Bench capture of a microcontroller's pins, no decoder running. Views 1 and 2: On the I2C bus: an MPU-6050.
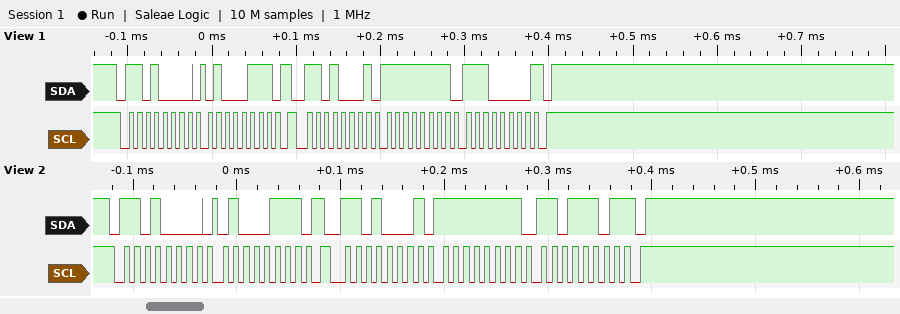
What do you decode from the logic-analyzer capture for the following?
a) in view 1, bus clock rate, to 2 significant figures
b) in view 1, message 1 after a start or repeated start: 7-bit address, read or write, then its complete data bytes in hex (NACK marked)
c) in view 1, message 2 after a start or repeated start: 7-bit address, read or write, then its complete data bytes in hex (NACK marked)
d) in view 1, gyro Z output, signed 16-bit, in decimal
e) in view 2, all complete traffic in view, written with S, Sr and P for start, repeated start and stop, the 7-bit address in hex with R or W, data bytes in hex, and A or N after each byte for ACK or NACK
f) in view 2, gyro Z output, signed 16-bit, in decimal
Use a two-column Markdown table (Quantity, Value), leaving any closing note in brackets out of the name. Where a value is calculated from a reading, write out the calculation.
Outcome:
| Quantity | Value |
|---|---|
| in view 1, bus clock rate, to 2 significant figures | 100 kHz |
| in view 1, message 1 after a start or repeated start: 7-bit address, read or write, then its complete data bytes in hex | 0x68 write: 47 |
| in view 1, message 2 after a start or repeated start: 7-bit address, read or write, then its complete data bytes in hex | 0x68 read: FF E0 NACK |
| in view 1, gyro Z output, signed 16-bit, in decimal | 0xFFE0 = -32 |
| in view 2, all complete traffic in view, written with S, Sr and P for start, repeated start and stop, the 7-bit address in hex with R or W, data bytes in hex, and A or N after each byte for ACK or NACK | S 68W A 47 A Sr 68R A FF A DD N P |
| in view 2, gyro Z output, signed 16-bit, in decimal | 0xFFDD = -35 |
